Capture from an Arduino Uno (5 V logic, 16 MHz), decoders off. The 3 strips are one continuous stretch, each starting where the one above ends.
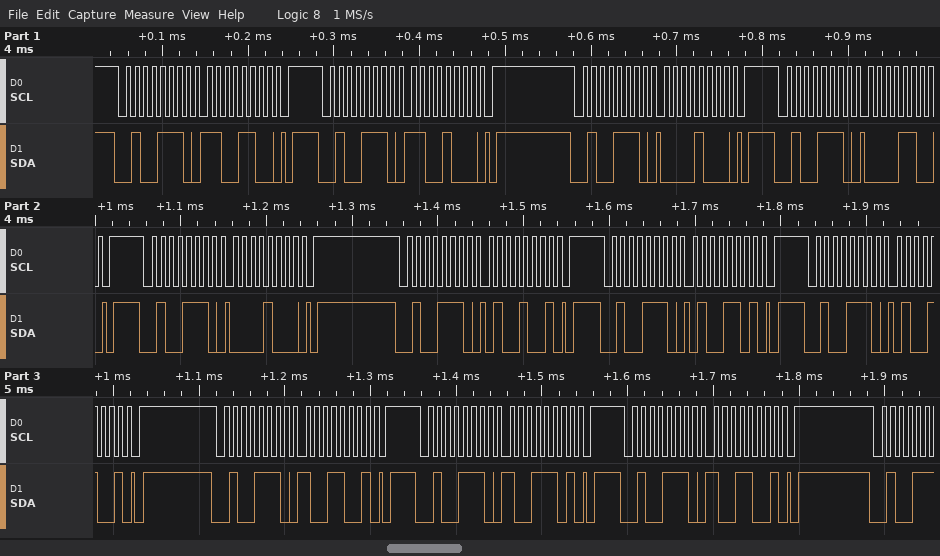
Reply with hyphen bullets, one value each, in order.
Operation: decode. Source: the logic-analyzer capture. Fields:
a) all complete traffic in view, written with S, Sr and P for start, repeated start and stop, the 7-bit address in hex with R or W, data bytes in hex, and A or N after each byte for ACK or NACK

- S 27W A CC A P S 27W A C8 A P S 27W A 08 A P S 27W A 0C A P S 27W A 08 A P S 27W A 49 A P S 27W A 4D A P S 27W A 49 A P S 27W A 99 A P S 27W A 9D A P S 27W A 99 A P
